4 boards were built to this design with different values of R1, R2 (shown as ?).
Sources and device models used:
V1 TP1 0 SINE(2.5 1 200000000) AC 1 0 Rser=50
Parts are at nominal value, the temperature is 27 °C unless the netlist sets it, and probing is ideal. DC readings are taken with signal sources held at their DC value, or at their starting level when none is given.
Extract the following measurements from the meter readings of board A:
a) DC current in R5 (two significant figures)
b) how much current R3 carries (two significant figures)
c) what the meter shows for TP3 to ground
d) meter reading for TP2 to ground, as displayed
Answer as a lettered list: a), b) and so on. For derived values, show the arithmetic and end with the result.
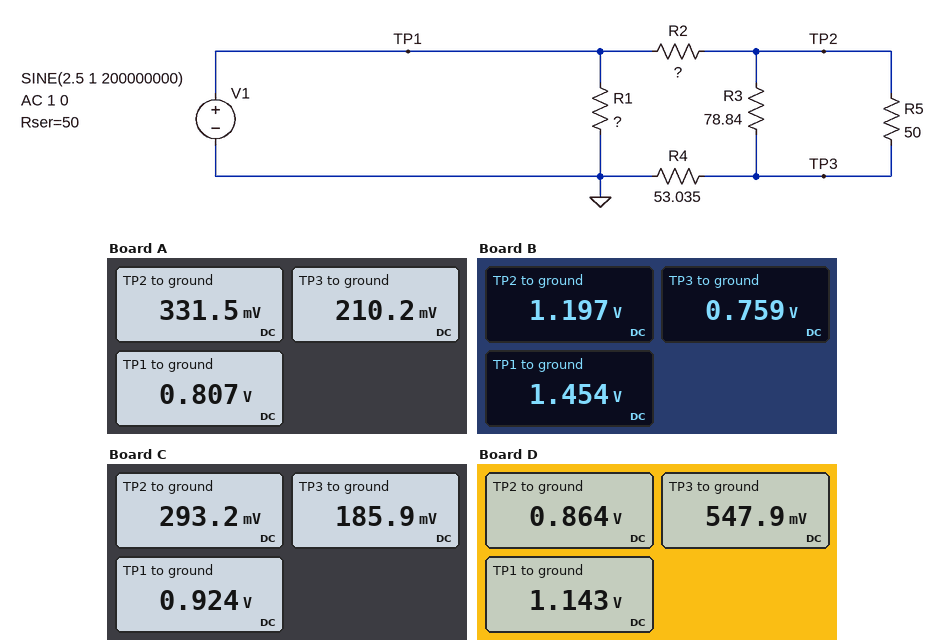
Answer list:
a) (331.5 mV - 210.2 mV) / 50 Ω = 2.4 mA
b) (331.5 mV - 210.2 mV) / 78.84 Ω = 1.5 mA
c) 210.2 mV
d) 331.5 mV
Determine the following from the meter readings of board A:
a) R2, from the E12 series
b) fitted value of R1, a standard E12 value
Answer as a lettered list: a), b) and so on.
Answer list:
a) 120 Ω
b) 27 Ω
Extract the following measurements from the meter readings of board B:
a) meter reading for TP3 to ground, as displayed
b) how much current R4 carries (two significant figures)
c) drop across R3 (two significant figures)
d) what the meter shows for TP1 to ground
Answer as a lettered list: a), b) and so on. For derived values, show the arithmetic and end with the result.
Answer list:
a) 0.759 V
b) (759 mV) / 53.03 Ω = 14 mA
c) 1.197 V - 759 mV = 440 mV
d) 1.454 V
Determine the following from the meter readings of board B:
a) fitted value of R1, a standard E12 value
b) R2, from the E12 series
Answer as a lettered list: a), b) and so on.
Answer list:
a) 220 Ω
b) 18 Ω
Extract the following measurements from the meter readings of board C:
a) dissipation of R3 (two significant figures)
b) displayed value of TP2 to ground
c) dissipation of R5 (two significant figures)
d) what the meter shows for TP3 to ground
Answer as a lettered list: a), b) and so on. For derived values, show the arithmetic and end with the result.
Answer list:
a) (293.2 mV - 185.9 mV)^2 / 78.84 Ω = 150 µW
b) 293.2 mV
c) (293.2 mV - 185.9 mV)^2 / 50 Ω = 230 µW
d) 185.9 mV
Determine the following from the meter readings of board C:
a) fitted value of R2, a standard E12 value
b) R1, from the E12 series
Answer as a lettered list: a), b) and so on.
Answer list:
a) 180 Ω
b) 33 Ω
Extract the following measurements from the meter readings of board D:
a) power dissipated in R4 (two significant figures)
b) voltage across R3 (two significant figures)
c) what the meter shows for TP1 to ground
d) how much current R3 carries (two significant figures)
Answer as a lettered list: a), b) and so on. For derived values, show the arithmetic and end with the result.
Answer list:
a) (547.9 mV)^2 / 53.03 Ω = 5.7 mW
b) 864 mV - 547.9 mV = 320 mV
c) 1.143 V
d) (864 mV - 547.9 mV) / 78.84 Ω = 4.0 mA
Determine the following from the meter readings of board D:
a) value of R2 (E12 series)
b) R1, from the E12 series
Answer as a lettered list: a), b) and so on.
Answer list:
a) 27 Ω
b) 68 Ω
